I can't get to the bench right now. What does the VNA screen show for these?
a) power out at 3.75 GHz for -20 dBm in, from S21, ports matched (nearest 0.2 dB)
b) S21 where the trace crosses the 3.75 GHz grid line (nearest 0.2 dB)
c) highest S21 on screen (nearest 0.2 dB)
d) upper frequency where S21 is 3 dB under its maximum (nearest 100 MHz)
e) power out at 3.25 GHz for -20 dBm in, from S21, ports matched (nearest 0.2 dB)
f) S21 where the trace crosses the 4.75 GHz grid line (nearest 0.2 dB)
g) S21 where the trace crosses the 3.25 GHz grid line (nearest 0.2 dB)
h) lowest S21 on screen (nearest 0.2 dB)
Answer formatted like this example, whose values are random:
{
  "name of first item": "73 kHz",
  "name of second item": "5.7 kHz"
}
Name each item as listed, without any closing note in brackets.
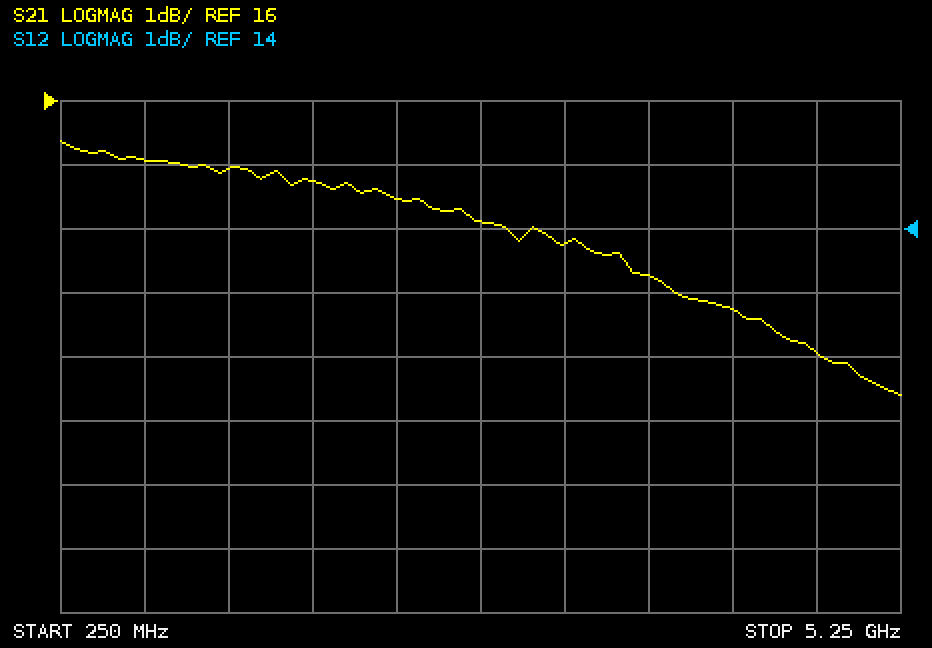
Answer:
{
  "power out at 3.75 GHz for -20 dBm in, from S21, ports matched": "-6.8 dBm",
  "S21 where the trace crosses the 3.75 GHz grid line": "13.2 dB",
  "highest S21 on screen": "15.4 dB",
  "upper frequency where S21 is 3 dB under its maximum": "4.5 GHz",
  "power out at 3.25 GHz for -20 dBm in, from S21, ports matched": "-6.2 dBm",
  "S21 where the trace crosses the 4.75 GHz grid line": "12.0 dB",
  "S21 where the trace crosses the 3.25 GHz grid line": "13.8 dB",
  "lowest S21 on screen": "11.4 dB"
}
